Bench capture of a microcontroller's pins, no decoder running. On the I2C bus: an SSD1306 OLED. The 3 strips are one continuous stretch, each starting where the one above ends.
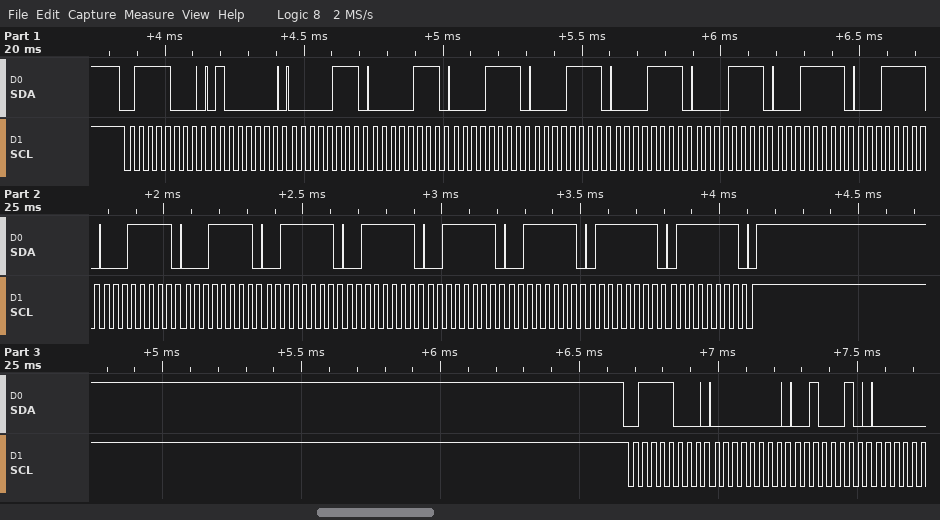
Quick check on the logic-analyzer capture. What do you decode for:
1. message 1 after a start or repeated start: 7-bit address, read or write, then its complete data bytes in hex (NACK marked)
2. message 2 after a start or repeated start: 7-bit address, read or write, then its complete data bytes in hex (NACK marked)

0x3C write: 40 07 07 0F 0F 0F 0F 1F 1F 1F 1F 3F 3F 3F 3F 7F 7F
0x3C write: 00 22
